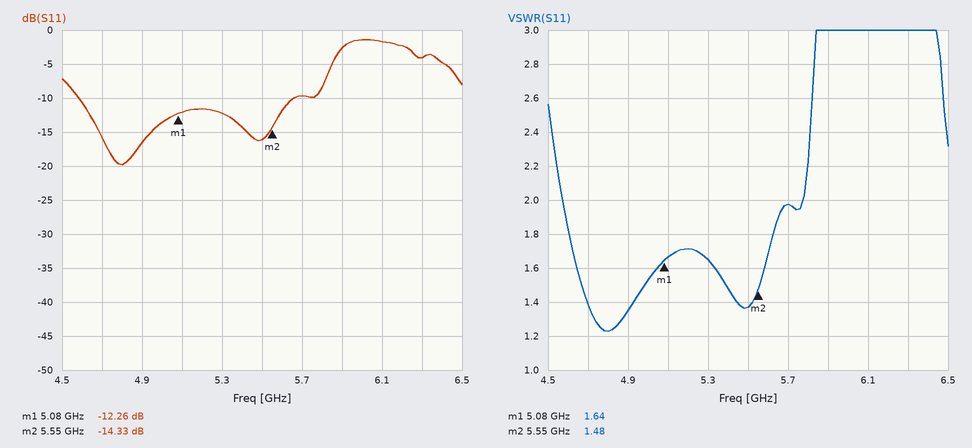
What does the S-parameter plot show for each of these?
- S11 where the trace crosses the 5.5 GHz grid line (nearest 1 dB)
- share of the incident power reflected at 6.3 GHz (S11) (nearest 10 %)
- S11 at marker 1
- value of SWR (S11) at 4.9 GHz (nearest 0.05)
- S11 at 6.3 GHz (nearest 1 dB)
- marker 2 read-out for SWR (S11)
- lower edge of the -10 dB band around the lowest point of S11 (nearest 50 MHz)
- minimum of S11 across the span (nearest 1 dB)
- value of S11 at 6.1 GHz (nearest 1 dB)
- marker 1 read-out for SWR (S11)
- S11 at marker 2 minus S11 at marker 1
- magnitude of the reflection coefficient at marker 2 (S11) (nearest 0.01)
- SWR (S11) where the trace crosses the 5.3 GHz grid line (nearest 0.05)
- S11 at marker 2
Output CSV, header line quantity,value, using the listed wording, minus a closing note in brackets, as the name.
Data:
quantity,value
S11 where the trace crosses the 5.5 GHz grid line,-16 dB
share of the incident power reflected at 6.3 GHz (S11),40 %
S11 at marker 1,-12.26 dB
value of SWR (S11) at 4.9 GHz,1.35
S11 at 6.3 GHz,-4 dB
marker 2 read-out for SWR,1.48
lower edge of the -10 dB band around the lowest point of S11,4.60 GHz
minimum of S11 across the span,-20 dB
value of S11 at 6.1 GHz,-2 dB
marker 1 read-out for SWR,1.64
S11 at marker 2 minus S11 at marker 1,-2.07 dB
magnitude of the reflection coefficient at marker 2 (S11),0.19
SWR (S11) where the trace crosses the 5.3 GHz grid line,1.65
S11 at marker 2,-14.33 dB
